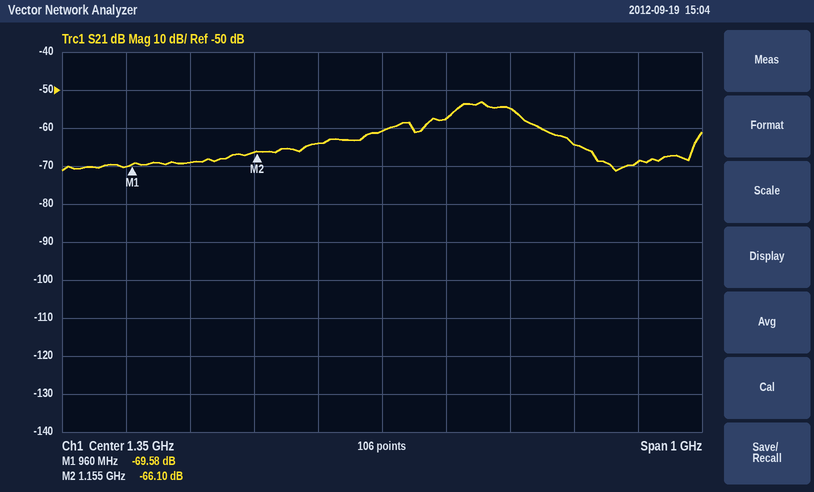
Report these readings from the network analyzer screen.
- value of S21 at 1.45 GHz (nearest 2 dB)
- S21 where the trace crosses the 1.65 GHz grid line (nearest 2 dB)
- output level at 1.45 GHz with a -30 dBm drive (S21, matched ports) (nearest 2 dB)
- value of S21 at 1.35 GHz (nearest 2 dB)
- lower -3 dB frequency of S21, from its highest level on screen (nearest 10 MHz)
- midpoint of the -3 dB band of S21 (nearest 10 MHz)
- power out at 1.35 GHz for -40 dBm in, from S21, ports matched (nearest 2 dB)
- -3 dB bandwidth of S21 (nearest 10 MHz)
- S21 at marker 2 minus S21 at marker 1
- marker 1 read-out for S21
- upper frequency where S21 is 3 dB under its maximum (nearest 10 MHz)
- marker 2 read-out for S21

-58 dB
-64 dB
-88 dBm
-60 dB
1.46 GHz
1.51 GHz
-100 dBm
100 MHz
3.48 dB
-69.58 dB
1.56 GHz
-66.10 dB
